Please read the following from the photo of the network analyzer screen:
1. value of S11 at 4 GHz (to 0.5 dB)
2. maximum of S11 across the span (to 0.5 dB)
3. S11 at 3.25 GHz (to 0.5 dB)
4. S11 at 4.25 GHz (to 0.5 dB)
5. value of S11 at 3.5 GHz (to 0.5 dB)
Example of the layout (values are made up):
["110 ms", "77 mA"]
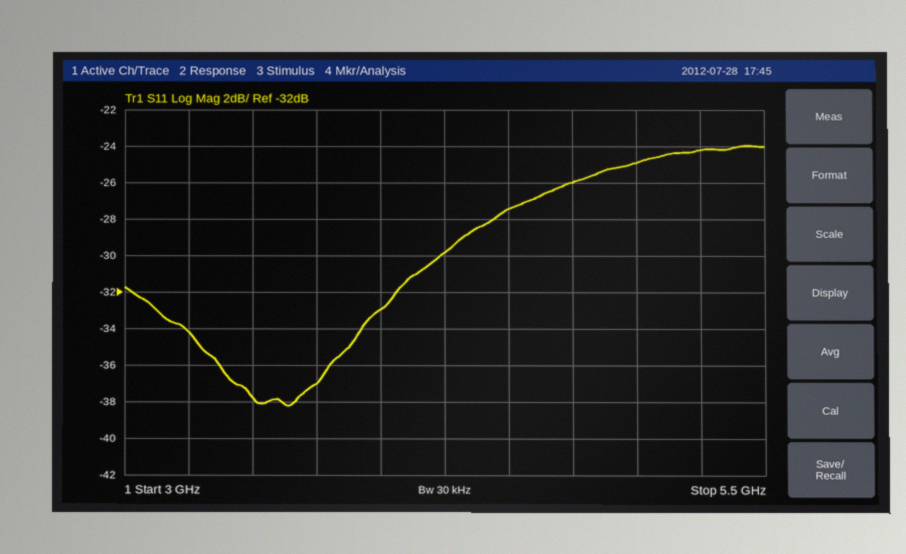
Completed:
["-33.0 dB", "-24.0 dB", "-34.0 dB", "-30.0 dB", "-38.0 dB"]
